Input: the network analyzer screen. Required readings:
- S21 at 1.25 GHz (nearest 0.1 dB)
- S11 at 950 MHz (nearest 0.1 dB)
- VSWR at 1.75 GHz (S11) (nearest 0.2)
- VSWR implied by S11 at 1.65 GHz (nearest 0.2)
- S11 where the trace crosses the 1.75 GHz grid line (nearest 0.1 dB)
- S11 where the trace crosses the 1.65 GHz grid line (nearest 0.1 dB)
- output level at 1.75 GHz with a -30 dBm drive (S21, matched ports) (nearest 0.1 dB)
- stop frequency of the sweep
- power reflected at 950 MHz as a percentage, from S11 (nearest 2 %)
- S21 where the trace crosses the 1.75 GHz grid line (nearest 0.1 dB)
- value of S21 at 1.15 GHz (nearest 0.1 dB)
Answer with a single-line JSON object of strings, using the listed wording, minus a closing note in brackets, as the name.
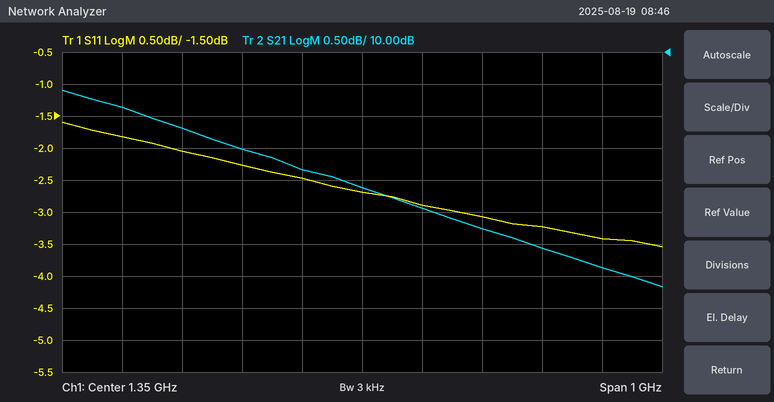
{"S21 at 1.25 GHz": "8.2 dB", "S11 at 950 MHz": "-1.8 dB", "VSWR at 1.75 GHz (S11)": "5.2", "VSWR implied by S11 at 1.65 GHz": "5.4", "S11 where the trace crosses the 1.75 GHz grid line": "-3.4 dB", "S11 where the trace crosses the 1.65 GHz grid line": "-3.2 dB", "output level at 1.75 GHz with a -30 dBm drive (S21, matched ports)": "-23.4 dBm", "stop frequency of the sweep": "1.85 GHz", "power reflected at 950 MHz as a percentage, from S11": "66 %", "S21 where the trace crosses the 1.75 GHz grid line": "6.6 dB", "value of S21 at 1.15 GHz": "8.5 dB"}
